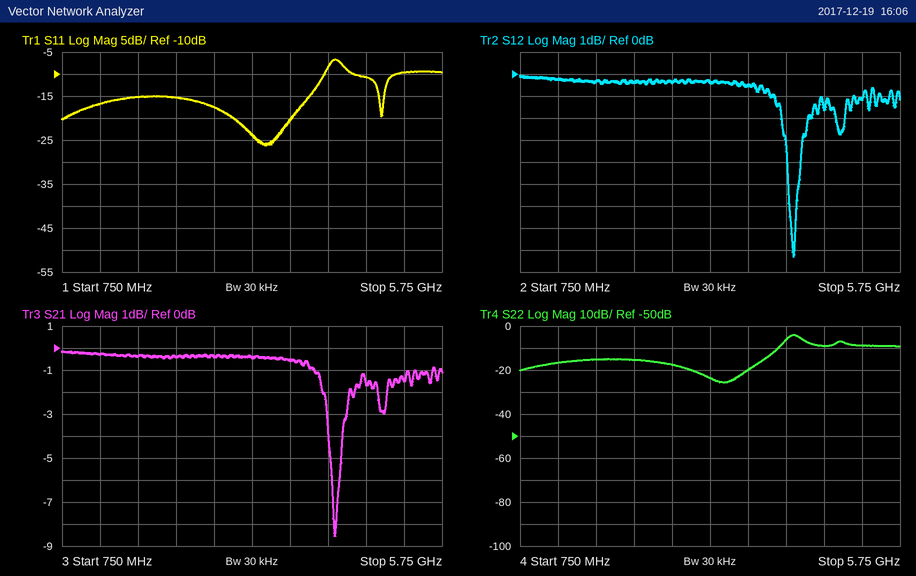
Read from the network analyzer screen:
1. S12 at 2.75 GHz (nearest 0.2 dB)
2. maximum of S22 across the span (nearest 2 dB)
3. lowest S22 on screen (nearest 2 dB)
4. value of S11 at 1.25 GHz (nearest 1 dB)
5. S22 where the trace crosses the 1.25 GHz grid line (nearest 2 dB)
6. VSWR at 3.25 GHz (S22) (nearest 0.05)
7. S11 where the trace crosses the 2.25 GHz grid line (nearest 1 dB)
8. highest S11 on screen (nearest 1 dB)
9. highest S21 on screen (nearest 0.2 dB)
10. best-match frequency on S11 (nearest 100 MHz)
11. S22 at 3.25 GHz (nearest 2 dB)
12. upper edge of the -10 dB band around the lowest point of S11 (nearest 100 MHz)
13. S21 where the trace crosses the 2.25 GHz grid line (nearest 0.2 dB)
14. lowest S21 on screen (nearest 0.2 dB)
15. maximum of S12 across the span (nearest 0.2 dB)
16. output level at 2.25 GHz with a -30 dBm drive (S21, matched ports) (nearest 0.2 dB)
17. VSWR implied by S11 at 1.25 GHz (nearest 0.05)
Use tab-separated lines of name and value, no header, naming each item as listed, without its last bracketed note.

S12 at 2.75 GHz	-0.4 dB
maximum of S22 across the span	-4 dB
lowest S22 on screen	-26 dB
value of S11 at 1.25 GHz	-17 dB
S22 where the trace crosses the 1.25 GHz grid line	-16 dB
VSWR at 3.25 GHz (S22)	1.15
S11 where the trace crosses the 2.25 GHz grid line	-15 dB
highest S11 on screen	-7 dB
highest S21 on screen	-0.2 dB
best-match frequency on S11	3.4 GHz
S22 at 3.25 GHz	-24 dB
upper edge of the -10 dB band around the lowest point of S11	4.2 GHz
S21 where the trace crosses the 2.25 GHz grid line	-0.4 dB
lowest S21 on screen	-8.6 dB
maximum of S12 across the span	0.0 dB
output level at 2.25 GHz with a -30 dBm drive (S21, matched ports)	-30.4 dBm
VSWR implied by S11 at 1.25 GHz	1.35
